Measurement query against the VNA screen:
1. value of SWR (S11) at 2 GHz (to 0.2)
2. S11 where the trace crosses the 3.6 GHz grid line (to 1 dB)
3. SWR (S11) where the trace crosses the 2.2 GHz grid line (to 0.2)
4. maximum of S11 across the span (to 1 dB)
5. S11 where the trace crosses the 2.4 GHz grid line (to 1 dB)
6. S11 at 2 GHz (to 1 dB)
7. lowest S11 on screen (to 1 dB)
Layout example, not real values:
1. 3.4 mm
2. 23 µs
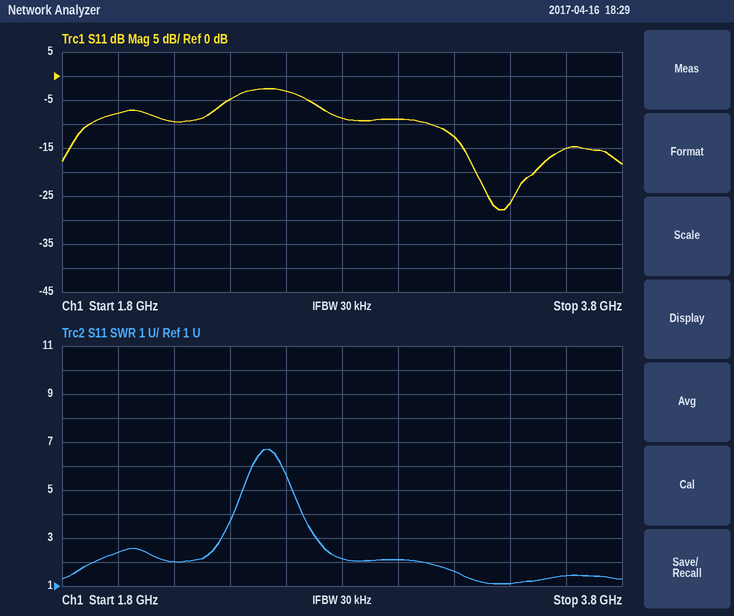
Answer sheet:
1. 2.4
2. -15 dB
3. 2.0
4. -3 dB
5. -5 dB
6. -8 dB
7. -28 dB
